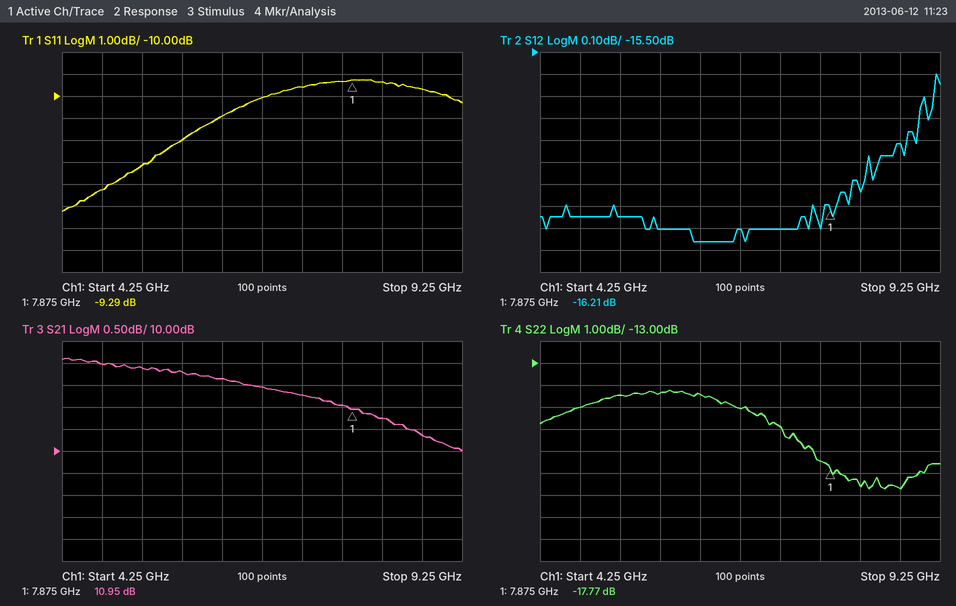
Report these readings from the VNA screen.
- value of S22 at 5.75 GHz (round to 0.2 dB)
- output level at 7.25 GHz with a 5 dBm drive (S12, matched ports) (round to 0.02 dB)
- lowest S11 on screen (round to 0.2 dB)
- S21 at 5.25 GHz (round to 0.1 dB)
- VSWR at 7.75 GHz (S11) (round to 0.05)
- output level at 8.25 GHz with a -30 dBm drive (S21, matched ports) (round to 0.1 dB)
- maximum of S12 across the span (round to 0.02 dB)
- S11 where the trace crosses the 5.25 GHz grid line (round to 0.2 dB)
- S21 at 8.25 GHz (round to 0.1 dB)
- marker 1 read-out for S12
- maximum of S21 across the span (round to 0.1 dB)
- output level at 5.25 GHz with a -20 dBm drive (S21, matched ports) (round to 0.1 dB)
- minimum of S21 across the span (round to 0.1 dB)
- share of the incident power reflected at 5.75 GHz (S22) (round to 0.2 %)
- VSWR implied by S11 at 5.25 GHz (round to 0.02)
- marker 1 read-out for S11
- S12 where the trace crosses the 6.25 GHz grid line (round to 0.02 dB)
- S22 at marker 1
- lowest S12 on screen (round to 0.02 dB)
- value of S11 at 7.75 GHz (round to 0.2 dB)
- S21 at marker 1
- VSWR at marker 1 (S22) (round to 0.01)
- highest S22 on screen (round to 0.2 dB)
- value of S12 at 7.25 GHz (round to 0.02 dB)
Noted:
-14.4 dB
-11.30 dBm
-15.2 dB
11.9 dB
2.05
-19.3 dBm
-15.60 dB
-13.2 dB
10.7 dB
-16.21 dB
12.1 dB
-8.1 dBm
10.0 dB
3.6 %
1.56
-9.29 dB
-16.36 dB
-17.77 dB
-16.36 dB
-9.4 dB
10.95 dB
1.30
-14.2 dB
-16.30 dB
